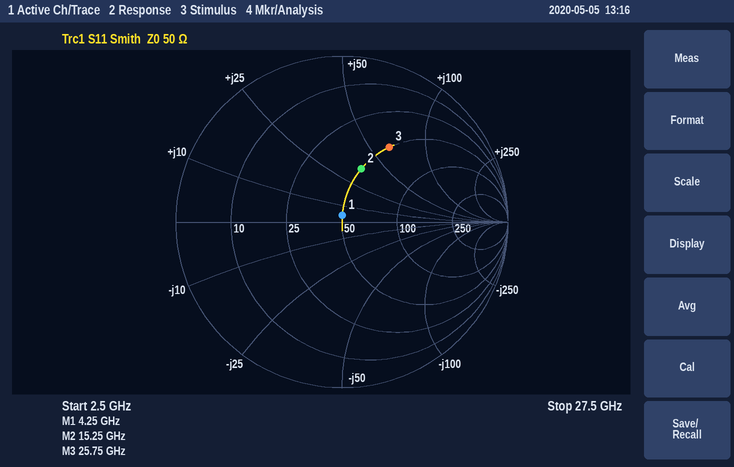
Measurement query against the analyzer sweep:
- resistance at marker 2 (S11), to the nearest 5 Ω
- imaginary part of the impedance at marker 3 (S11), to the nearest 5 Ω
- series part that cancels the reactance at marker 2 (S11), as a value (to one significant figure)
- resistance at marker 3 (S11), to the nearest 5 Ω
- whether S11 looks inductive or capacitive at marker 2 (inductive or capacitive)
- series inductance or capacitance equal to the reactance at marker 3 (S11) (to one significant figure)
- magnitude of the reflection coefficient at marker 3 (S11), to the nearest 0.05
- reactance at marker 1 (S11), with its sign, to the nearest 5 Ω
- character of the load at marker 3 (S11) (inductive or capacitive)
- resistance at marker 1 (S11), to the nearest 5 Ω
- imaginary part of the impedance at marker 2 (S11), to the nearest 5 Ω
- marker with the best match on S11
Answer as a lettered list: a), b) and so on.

a) 50 Ω
b) +65 Ω
c) 300 fF
d) 50 Ω
e) inductive
f) 400 pH
g) 0.55
h) +5 Ω
i) inductive
j) 50 Ω
k) +35 Ω
l) marker 1
